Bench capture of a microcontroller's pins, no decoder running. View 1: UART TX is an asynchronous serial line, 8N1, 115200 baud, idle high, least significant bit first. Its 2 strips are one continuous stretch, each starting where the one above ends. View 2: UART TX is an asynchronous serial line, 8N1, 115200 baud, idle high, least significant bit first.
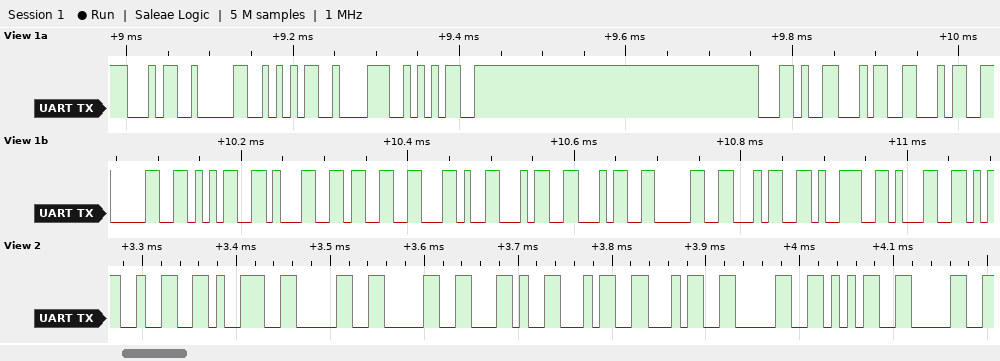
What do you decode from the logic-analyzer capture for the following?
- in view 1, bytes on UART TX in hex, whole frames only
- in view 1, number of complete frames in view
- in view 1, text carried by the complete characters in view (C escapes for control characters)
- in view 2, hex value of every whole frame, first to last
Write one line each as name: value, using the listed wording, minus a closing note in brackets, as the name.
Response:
in view 1, bytes on UART TX in hex, whole frames only: 0x34 0x30 0x35 0x38 0x35 0x2C 0x34 0x34 0x30 0x35 0x31 0x33 0x2C 0x34 0x34 0x30 0x34 0x39 0x31
in view 1, number of complete frames in view: 19
in view 1, text carried by the complete characters in view: "40585,440513,440491"
in view 2, hex value of every whole frame, first to last: 32 39 30 30 2C 34 34 30 35 30
